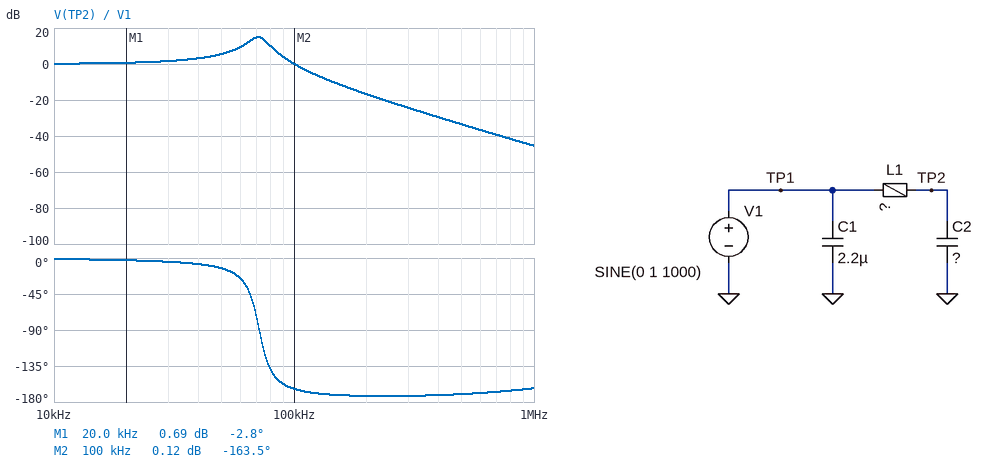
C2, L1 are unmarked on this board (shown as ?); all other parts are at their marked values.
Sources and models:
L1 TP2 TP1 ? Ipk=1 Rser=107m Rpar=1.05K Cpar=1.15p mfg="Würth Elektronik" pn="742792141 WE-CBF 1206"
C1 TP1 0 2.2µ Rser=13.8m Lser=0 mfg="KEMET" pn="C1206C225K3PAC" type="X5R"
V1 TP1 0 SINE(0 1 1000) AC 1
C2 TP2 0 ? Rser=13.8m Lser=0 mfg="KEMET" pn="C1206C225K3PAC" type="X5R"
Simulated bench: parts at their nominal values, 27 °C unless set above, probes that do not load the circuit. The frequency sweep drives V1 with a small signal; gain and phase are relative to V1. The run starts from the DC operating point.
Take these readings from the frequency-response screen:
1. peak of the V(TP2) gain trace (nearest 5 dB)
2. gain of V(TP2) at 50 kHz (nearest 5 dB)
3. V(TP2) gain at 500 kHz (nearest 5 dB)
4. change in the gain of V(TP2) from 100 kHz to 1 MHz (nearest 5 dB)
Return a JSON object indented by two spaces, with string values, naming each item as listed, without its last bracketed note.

{
  "peak of the V(TP2) gain trace": "15 dB",
  "gain of V(TP2) at 50 kHz": "5 dB",
  "V(TP2) gain at 500 kHz": "-35 dB",
  "change in the gain of V(TP2) from 100 kHz to 1 MHz": "-45 dB"
}
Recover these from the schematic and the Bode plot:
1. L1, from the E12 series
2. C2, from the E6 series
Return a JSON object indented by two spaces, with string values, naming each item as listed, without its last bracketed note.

{
  "L1, from the E12 series": "1.5 µH",
  "C2, from the E6 series": "3.3 µF"
}
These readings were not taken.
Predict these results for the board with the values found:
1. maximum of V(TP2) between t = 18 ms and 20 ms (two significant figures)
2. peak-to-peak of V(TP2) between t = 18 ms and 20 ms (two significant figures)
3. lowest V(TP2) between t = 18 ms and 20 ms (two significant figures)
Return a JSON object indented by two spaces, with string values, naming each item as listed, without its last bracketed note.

{
  "maximum of V(TP2) between t = 18 ms and 20 ms": "1.0 V",
  "peak-to-peak of V(TP2) between t = 18 ms and 20 ms": "2.0 V",
  "lowest V(TP2) between t = 18 ms and 20 ms": "-1.0 V"
}
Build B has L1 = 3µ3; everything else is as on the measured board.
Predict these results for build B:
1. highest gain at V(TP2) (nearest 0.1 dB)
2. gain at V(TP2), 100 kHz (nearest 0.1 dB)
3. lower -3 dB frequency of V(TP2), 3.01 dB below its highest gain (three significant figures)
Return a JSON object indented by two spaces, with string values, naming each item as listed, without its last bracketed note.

{
  "highest gain at V(TP2)": "18.3 dB",
  "gain at V(TP2), 100 kHz": "-10.4 dB",
  "lower -3 dB frequency of V(TP2), 3.01 dB below its highest gain": "45.0 kHz"
}
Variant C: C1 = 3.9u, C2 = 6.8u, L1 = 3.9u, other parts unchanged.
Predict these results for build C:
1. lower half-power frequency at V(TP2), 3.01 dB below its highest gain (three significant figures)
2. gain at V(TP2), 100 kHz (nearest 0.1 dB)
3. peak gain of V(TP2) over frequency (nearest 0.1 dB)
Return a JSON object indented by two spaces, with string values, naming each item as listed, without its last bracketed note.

{
  "lower half-power frequency at V(TP2), 3.01 dB below its highest gain": "28.1 kHz",
  "gain at V(TP2), 100 kHz": "-19.5 dB",
  "peak gain of V(TP2) over frequency": "15.9 dB"
}
